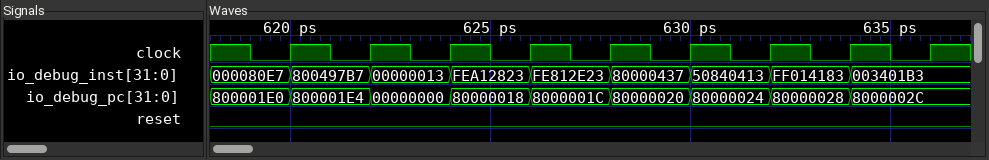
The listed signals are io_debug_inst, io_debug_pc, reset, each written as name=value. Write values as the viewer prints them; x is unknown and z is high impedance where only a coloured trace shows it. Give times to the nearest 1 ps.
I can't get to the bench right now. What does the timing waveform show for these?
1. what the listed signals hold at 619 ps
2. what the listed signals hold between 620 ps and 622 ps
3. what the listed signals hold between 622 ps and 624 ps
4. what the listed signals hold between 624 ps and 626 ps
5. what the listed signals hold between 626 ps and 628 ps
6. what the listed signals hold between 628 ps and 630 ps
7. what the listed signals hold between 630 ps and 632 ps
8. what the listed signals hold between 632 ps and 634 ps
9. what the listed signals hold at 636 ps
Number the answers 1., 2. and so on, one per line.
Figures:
1. io_debug_inst=000080E7, io_debug_pc=800001E0, reset=0
2. io_debug_inst=800497B7, io_debug_pc=800001E4, reset=0
3. io_debug_inst=00000013, io_debug_pc=00000000, reset=0
4. io_debug_inst=FEA12823, io_debug_pc=80000018, reset=0
5. io_debug_inst=FE812E23, io_debug_pc=8000001C, reset=0
6. io_debug_inst=80000437, io_debug_pc=80000020, reset=0
7. io_debug_inst=50840413, io_debug_pc=80000024, reset=0
8. io_debug_inst=FF014183, io_debug_pc=80000028, reset=0
9. io_debug_inst=003401B3, io_debug_pc=8000002C, reset=0
